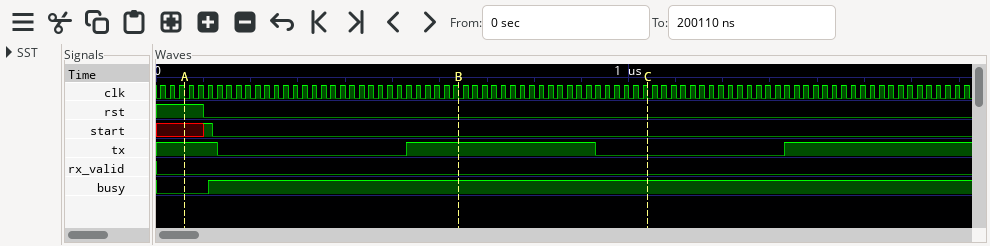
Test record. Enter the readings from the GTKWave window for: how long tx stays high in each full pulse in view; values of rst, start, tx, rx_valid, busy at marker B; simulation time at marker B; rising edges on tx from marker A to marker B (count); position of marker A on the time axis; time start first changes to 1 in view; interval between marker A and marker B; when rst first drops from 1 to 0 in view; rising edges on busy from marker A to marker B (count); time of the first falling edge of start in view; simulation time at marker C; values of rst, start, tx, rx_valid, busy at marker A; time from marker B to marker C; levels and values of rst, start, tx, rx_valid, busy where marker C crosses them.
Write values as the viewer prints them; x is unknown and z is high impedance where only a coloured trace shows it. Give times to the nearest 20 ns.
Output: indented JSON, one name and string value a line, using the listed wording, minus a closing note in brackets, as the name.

{
  "how long tx stays high in each full pulse in view": "400 ns",
  "values of rst, start, tx, rx_valid, busy at marker B": "rst=0, start=0, tx=1, rx_valid=0, busy=1",
  "simulation time at marker B": "640 ns",
  "rising edges on tx from marker A to marker B": "1",
  "position of marker A on the time axis": "60 ns",
  "time start first changes to 1 in view": "100 ns",
  "interval between marker A and marker B": "580 ns",
  "when rst first drops from 1 to 0 in view": "100 ns",
  "rising edges on busy from marker A to marker B": "1",
  "time of the first falling edge of start in view": "120 ns",
  "simulation time at marker C": "1040 ns",
  "values of rst, start, tx, rx_valid, busy at marker A": "rst=1, start=x, tx=1, rx_valid=0, busy=0",
  "time from marker B to marker C": "400 ns",
  "levels and values of rst, start, tx, rx_valid, busy where marker C crosses them": "rst=0, start=0, tx=0, rx_valid=0, busy=1"
}
